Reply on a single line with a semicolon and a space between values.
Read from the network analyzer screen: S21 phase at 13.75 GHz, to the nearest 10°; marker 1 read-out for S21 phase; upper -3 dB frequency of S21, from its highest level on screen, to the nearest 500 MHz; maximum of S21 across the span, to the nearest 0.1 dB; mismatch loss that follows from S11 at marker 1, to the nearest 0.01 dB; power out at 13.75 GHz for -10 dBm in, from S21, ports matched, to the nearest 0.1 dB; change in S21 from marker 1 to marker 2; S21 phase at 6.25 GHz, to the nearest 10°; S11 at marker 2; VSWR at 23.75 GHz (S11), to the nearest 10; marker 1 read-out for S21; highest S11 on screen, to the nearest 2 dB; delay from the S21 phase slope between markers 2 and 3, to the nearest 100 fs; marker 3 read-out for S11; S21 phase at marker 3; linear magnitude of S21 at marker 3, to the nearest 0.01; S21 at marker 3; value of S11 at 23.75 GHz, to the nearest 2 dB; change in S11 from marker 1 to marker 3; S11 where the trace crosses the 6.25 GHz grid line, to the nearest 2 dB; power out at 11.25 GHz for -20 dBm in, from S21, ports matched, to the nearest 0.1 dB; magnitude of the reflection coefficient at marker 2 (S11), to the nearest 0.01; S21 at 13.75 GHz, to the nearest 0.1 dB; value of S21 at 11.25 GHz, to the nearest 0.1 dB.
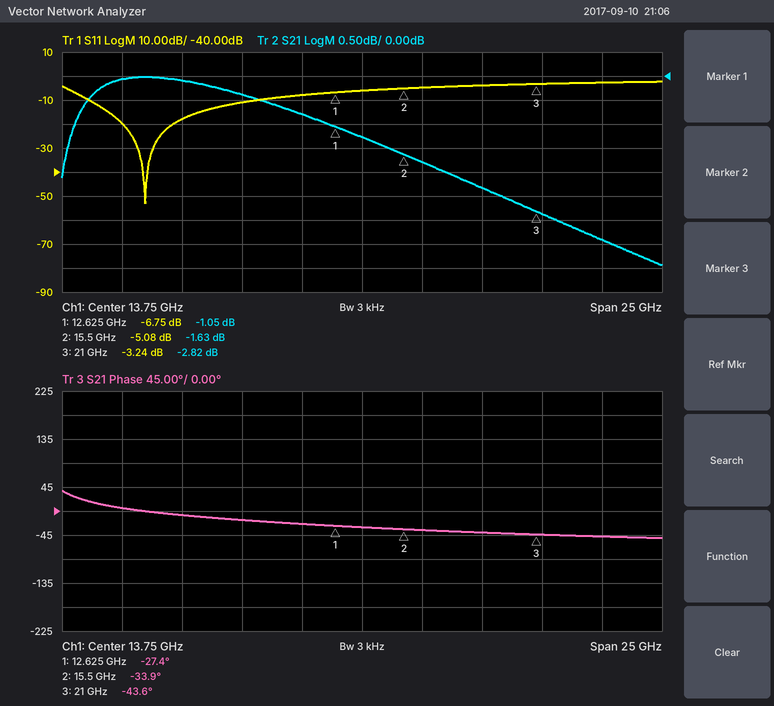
-30°; -27.4°; 22.0 GHz; 0.0 dB; 1.03 dB; -11.3 dBm; -0.58 dB; -10°; -5.08 dB; 10; -1.05 dB; -2 dB; 4.9 ps; -3.24 dB; -43.6°; 0.72; -2.82 dB; -2 dB; 3.51 dB; -18 dB; -20.8 dBm; 0.56; -1.3 dB; -0.8 dB
